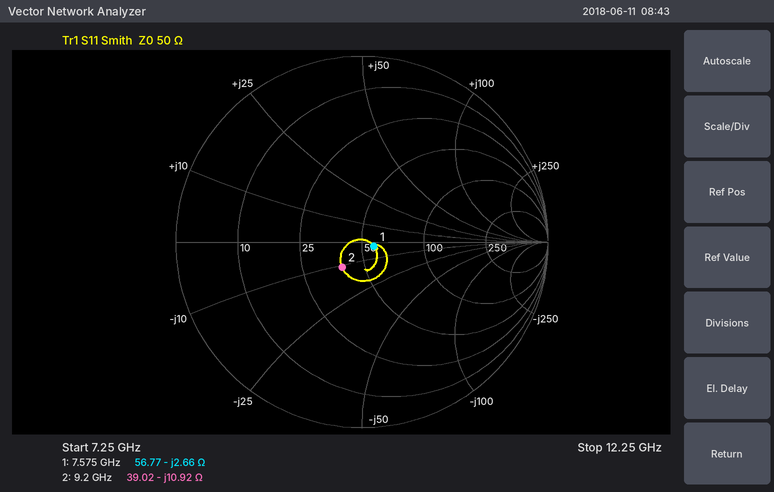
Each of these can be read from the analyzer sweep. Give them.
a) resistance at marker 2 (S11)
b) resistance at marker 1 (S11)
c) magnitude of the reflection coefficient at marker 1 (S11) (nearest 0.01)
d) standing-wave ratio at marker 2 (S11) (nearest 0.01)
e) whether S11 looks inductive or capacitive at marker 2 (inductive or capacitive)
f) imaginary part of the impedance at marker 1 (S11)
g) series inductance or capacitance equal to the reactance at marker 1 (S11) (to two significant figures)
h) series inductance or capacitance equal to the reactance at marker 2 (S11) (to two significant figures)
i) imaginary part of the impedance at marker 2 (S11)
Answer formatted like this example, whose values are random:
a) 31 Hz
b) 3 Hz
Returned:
a) 39.02 Ω
b) 56.77 Ω
c) 0.07
d) 1.42
e) capacitive
f) -2.66 Ω
g) 7.9 pF
h) 1.6 pF
i) -10.92 Ω
